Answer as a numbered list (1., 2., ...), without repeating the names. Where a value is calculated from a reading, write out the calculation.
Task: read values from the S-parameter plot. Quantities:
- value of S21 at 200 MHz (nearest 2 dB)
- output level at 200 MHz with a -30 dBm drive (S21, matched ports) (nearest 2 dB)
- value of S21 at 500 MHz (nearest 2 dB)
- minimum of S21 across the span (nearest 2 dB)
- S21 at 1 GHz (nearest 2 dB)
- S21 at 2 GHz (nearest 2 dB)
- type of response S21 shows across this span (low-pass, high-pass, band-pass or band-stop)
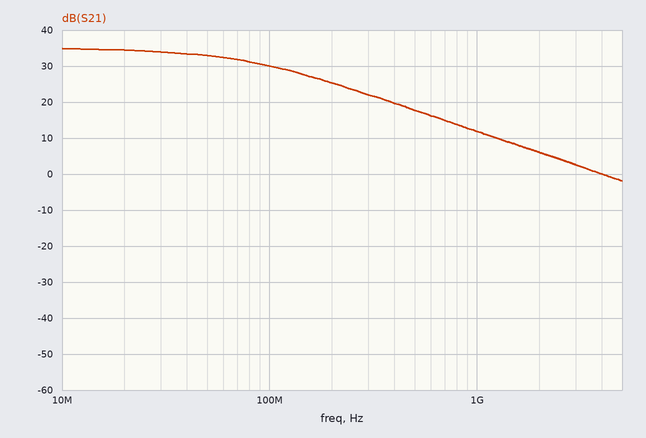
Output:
1. 26 dB
2. -30 dBm + (26 dB) = -4 dBm
3. 18 dB
4. -2 dB
5. 12 dB
6. 6 dB
7. low-pass
